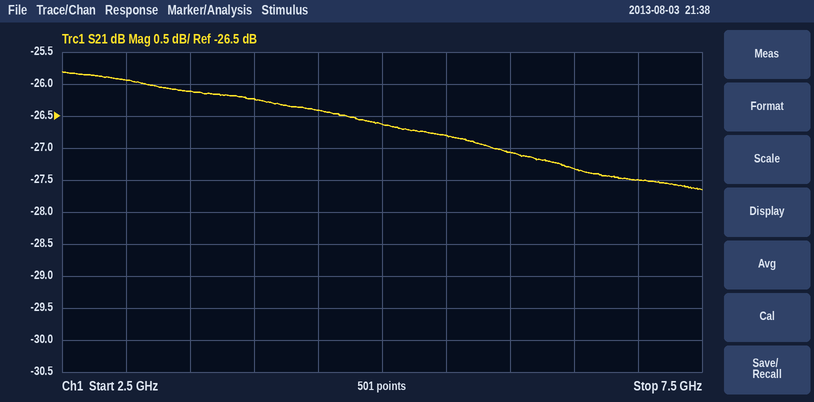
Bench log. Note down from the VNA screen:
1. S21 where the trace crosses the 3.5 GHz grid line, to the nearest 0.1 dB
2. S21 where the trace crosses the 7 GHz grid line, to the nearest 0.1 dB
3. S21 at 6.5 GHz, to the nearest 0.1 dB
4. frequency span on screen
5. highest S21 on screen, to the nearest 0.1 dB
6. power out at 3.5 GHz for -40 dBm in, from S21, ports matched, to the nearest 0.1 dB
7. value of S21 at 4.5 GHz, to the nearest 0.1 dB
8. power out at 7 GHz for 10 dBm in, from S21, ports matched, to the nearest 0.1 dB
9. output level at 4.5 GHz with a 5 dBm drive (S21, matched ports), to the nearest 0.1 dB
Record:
-26.1 dB
-27.5 dB
-27.3 dB
5 GHz
-25.8 dB
-66.1 dBm
-26.4 dB
-17.5 dBm
-21.4 dBm
